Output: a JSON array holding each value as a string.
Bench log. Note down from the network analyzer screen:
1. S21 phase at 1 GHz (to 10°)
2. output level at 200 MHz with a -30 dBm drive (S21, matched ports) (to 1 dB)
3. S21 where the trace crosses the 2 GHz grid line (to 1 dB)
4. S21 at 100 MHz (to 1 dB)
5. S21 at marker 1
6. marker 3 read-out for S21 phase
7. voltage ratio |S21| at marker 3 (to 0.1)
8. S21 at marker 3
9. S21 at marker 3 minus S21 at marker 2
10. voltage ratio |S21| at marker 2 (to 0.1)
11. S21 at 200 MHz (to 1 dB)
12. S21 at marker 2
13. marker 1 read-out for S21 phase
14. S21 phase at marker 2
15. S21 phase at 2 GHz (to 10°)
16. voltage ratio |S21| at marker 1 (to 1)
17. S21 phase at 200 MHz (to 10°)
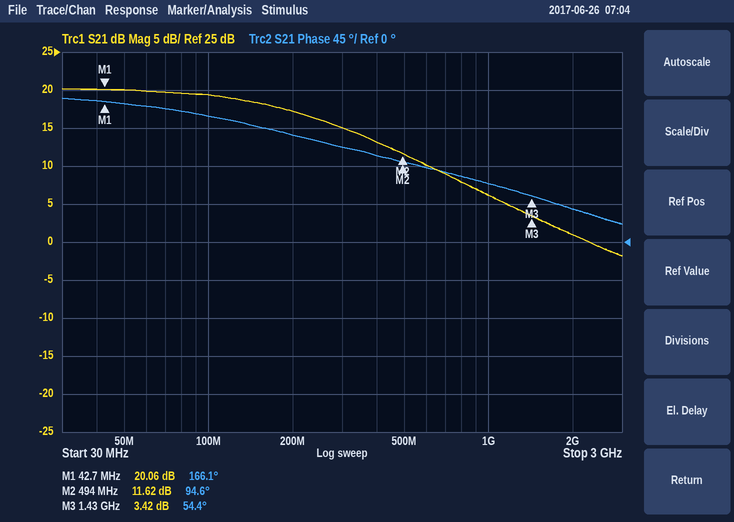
["70°", "-13 dBm", "1 dB", "19 dB", "20.06 dB", "54.4°", "1.5", "3.42 dB", "-8.20 dB", "3.8", "17 dB", "11.62 dB", "166.1°", "94.6°", "40°", "10", "130°"]
